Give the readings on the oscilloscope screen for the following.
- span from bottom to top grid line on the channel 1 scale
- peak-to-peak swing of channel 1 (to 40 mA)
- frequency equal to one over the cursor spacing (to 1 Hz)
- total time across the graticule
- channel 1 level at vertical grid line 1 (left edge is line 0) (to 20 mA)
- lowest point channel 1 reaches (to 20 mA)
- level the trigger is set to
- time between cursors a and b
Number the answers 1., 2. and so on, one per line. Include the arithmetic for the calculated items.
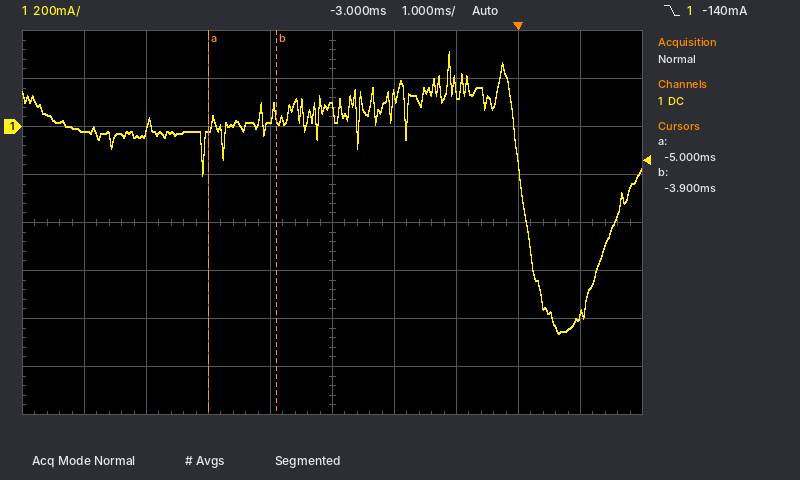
1. 1.6 A
2. 1.16 A
3. 1 / 1.1 ms ≈ 909 Hz
4. 10 ms
5. -20 mA
6. -860 mA
7. -140 mA
8. -3.9 ms − (-5 ms) = 1.1 ms
